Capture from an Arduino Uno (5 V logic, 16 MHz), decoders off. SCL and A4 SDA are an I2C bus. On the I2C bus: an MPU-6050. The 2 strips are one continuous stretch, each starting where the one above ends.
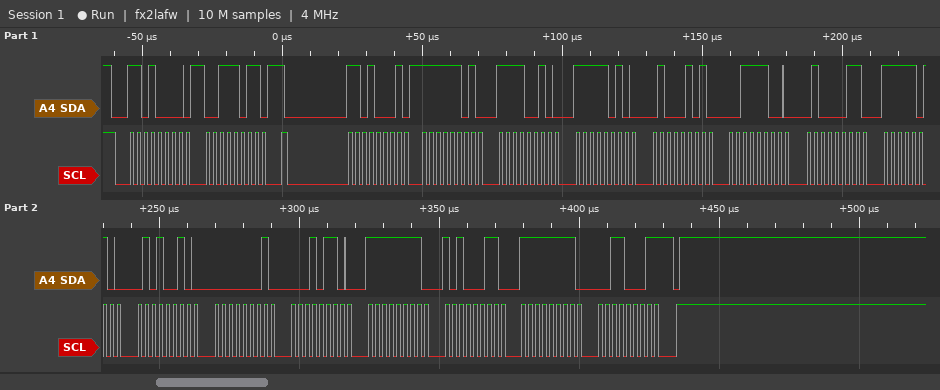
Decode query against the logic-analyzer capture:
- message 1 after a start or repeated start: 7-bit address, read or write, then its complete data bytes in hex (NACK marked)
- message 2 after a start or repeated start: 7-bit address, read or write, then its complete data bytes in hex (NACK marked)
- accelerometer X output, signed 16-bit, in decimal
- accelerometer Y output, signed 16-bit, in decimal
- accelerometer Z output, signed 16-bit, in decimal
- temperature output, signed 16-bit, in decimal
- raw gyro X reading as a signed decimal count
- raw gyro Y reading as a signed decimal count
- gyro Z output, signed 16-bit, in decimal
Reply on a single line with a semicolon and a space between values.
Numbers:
0x68 write: 3B; 0x68 read: FD F2 FA 45 3C 43 FA 52 01 16 FF A3 FF 31 NACK; -526; -1467; 15427; -1454; 278; -93; -207
